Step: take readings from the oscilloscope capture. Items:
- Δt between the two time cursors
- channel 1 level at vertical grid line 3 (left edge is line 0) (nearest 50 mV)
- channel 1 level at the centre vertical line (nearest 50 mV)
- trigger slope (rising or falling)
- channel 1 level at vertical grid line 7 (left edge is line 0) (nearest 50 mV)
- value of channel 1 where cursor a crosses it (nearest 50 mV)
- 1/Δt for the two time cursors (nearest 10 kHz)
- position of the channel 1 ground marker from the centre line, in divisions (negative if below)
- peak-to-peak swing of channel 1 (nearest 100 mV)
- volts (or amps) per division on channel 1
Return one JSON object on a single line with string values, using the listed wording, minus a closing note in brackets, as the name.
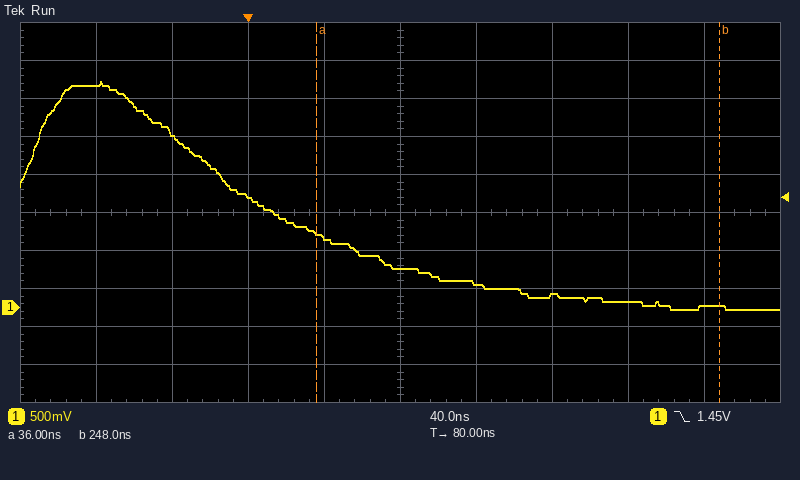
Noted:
{"Δt between the two time cursors": "212 ns", "channel 1 level at vertical grid line 3 (left edge is line 0)": "1.45 V", "channel 1 level at the centre vertical line": "500 mV", "trigger slope": "falling", "channel 1 level at vertical grid line 7 (left edge is line 0)": "150 mV", "value of channel 1 where cursor a crosses it": "1.00 V", "1/Δt for the two time cursors": "4.72 MHz", "position of the channel 1 ground marker from the centre line, in divisions": "-2.5 div", "peak-to-peak swing of channel 1": "3.00 V", "volts (or amps) per division on channel 1": "500 mV"}
